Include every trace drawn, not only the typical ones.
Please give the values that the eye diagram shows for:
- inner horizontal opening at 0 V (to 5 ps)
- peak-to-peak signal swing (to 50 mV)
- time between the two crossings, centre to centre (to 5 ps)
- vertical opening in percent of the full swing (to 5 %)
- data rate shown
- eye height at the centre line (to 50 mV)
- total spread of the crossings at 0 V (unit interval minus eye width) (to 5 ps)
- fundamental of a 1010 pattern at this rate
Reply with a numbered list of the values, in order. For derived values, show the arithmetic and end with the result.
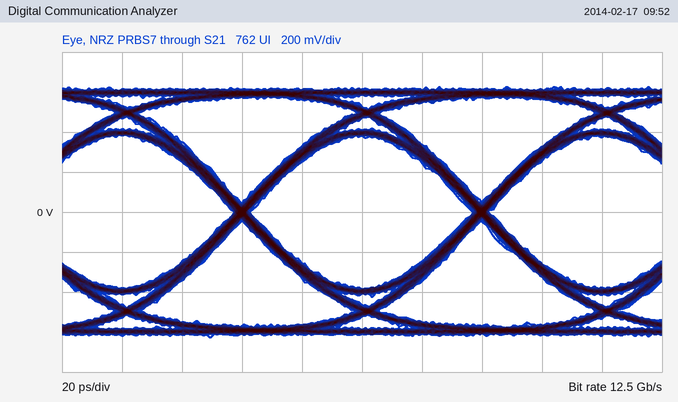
1. 75 ps
2. 1.25 V
3. 80 ps
4. 750 mV / 1.25 V ≈ 60 %
5. 12.5 Gb/s
6. 750 mV
7. 5 ps
8. 6.25 GHz
